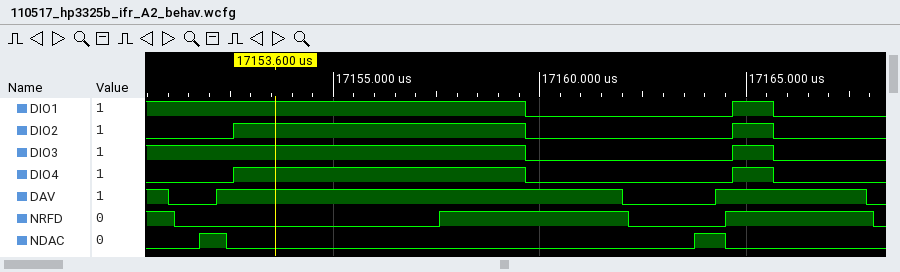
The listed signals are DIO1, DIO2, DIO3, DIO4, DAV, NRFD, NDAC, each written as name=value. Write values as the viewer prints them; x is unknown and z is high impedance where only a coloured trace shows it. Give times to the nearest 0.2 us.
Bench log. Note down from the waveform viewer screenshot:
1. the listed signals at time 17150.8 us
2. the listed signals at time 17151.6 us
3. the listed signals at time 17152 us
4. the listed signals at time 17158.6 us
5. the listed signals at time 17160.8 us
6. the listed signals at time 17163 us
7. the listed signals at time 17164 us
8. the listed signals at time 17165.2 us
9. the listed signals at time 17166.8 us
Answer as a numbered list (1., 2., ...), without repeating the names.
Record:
1. DIO1=1, DIO2=0, DIO3=1, DIO4=0, DAV=1, NRFD=1, NDAC=0
2. DIO1=1, DIO2=0, DIO3=1, DIO4=0, DAV=0, NRFD=0, NDAC=0
3. DIO1=1, DIO2=0, DIO3=1, DIO4=0, DAV=0, NRFD=0, NDAC=1
4. DIO1=1, DIO2=1, DIO3=1, DIO4=1, DAV=1, NRFD=1, NDAC=0
5. DIO1=0, DIO2=0, DIO3=0, DIO4=0, DAV=1, NRFD=1, NDAC=0
6. DIO1=0, DIO2=0, DIO3=0, DIO4=0, DAV=0, NRFD=0, NDAC=0
7. DIO1=0, DIO2=0, DIO3=0, DIO4=0, DAV=0, NRFD=0, NDAC=1
8. DIO1=1, DIO2=1, DIO3=1, DIO4=1, DAV=1, NRFD=1, NDAC=0
9. DIO1=0, DIO2=0, DIO3=0, DIO4=0, DAV=1, NRFD=1, NDAC=0
